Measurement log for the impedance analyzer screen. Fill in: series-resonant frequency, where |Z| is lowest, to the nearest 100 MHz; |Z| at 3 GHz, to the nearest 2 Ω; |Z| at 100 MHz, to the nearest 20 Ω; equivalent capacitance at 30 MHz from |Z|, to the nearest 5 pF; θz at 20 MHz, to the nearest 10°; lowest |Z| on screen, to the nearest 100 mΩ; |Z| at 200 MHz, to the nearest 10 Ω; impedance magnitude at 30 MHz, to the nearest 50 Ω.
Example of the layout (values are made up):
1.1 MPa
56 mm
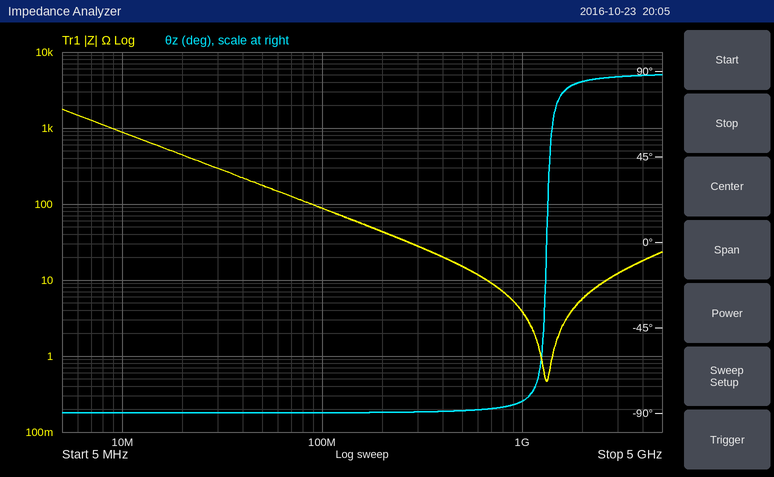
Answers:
1.3 GHz
12 Ω
80 Ω
20 pF
-90°
500 mΩ
40 Ω
300 Ω
